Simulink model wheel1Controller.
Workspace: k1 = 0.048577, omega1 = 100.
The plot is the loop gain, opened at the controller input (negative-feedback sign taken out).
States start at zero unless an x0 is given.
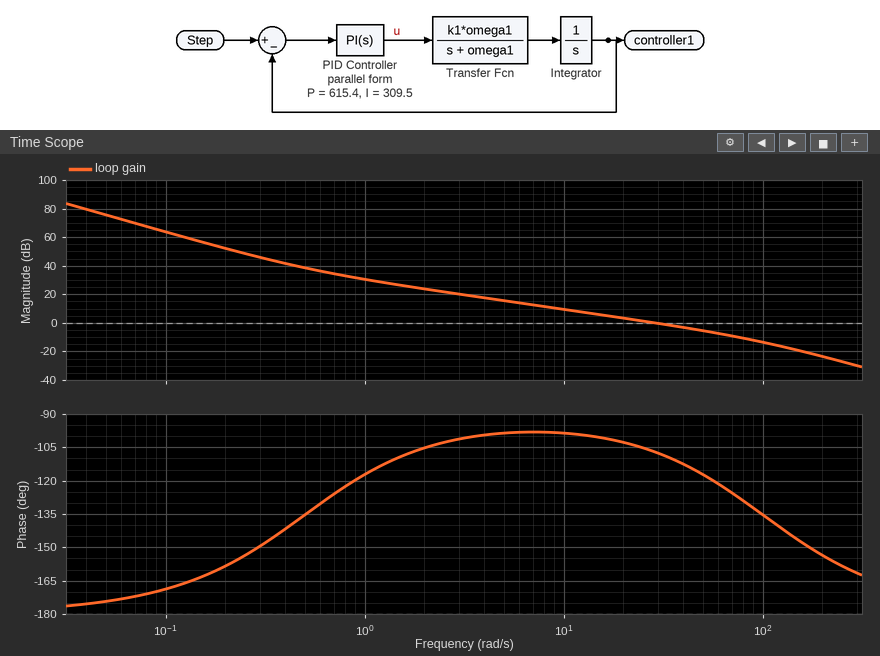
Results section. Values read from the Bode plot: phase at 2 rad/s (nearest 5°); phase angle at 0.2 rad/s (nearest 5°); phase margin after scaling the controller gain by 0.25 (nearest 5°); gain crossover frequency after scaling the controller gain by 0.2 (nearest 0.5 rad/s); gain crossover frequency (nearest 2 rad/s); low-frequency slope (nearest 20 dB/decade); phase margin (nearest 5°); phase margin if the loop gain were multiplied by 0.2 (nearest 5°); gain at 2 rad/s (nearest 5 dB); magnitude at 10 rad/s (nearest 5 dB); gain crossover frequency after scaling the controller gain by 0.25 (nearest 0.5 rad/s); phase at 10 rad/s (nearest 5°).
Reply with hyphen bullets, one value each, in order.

- -105°
- -160°
- 80°
- 6.0 rad/s
- 28 rad/s
- -40 dB/decade
- 75°
- 80°
- 25 dB
- 10 dB
- 7.5 rad/s
- -100°
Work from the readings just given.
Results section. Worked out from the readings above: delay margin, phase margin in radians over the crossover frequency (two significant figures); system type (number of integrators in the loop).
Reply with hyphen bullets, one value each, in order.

- 0.047 s
- 2
